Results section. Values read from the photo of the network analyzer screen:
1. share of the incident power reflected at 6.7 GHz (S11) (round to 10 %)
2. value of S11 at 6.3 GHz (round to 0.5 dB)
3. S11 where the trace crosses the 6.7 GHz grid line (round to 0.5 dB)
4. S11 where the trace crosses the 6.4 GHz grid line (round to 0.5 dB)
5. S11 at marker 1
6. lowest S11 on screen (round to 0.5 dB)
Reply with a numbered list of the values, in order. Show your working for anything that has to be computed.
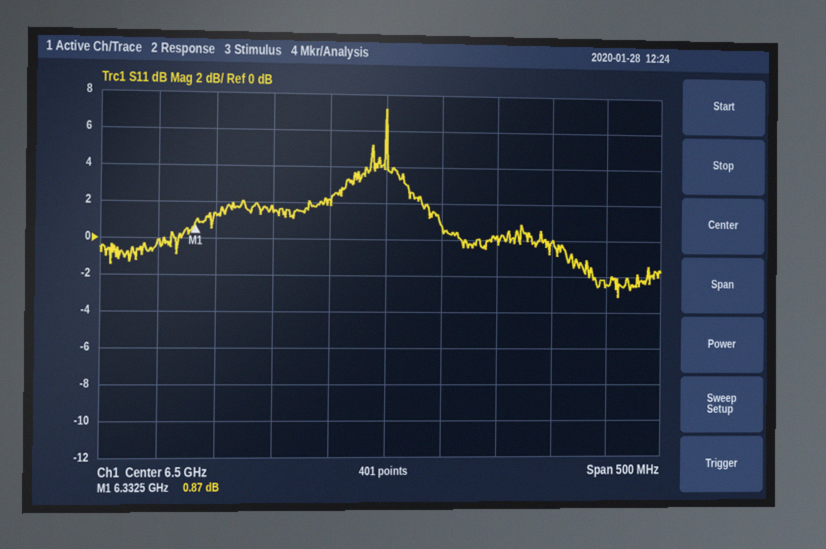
1. 10^(-2.5/10) ≈ 56.2 %, so 60 % to the nearest 10 %
2. 0.0 dB
3. -2.5 dB
4. 1.5 dB
5. 0.87 dB
6. -3.0 dB
